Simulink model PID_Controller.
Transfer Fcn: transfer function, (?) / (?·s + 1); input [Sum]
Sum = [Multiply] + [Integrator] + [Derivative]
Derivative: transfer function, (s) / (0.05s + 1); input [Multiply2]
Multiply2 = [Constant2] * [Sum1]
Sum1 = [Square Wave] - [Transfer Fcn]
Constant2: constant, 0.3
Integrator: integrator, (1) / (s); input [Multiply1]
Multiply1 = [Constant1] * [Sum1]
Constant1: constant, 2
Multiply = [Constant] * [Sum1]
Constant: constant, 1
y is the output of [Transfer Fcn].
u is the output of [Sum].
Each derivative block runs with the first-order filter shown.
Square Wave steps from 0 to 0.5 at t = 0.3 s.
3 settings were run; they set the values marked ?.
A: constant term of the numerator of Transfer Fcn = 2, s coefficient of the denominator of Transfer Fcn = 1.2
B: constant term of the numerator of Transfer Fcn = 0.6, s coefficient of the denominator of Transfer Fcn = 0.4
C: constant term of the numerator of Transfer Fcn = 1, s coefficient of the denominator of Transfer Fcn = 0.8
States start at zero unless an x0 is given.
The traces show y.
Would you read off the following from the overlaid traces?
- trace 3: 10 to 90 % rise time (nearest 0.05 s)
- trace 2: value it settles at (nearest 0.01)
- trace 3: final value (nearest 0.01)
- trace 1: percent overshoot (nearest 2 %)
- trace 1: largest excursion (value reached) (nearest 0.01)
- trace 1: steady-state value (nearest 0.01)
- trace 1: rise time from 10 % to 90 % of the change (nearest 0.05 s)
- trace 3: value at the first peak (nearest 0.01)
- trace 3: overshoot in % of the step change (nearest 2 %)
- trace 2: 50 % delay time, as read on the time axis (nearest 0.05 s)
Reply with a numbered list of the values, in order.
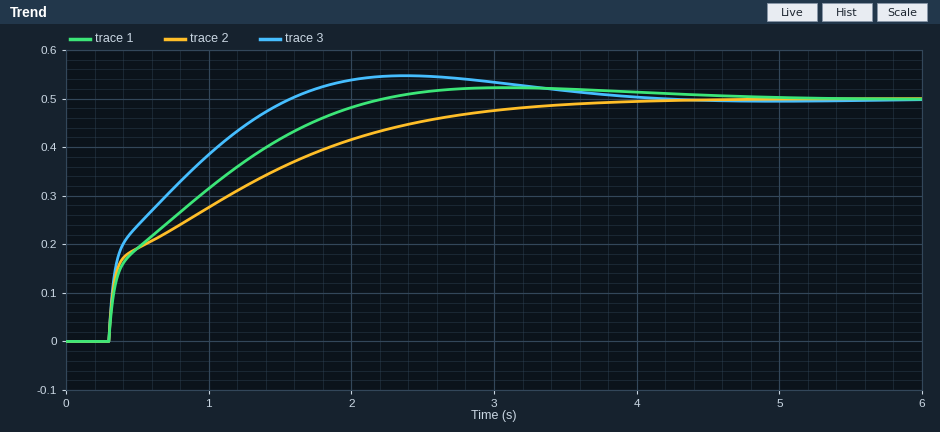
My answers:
1. 0.95 s
2. 0.50
3. 0.50
4. 4 %
5. 0.52
6. 0.50
7. 1.40 s
8. 0.55
9. 10 %
10. 0.85 s
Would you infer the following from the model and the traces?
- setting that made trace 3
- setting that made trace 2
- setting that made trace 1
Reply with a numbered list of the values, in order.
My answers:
1. A
2. B
3. C
